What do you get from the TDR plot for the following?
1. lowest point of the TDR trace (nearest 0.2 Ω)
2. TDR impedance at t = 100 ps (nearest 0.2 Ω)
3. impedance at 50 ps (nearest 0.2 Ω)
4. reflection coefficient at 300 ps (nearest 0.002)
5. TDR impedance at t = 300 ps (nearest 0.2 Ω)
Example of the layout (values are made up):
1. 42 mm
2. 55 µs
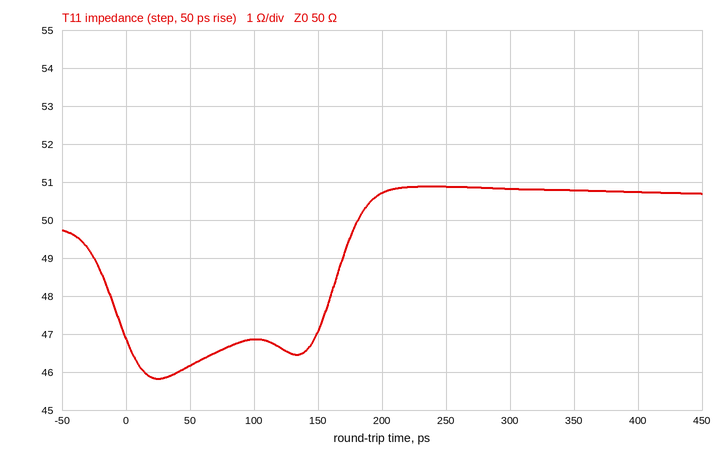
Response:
1. 45.8 Ω
2. 46.8 Ω
3. 46.2 Ω
4. +0.008
5. 50.8 Ω
